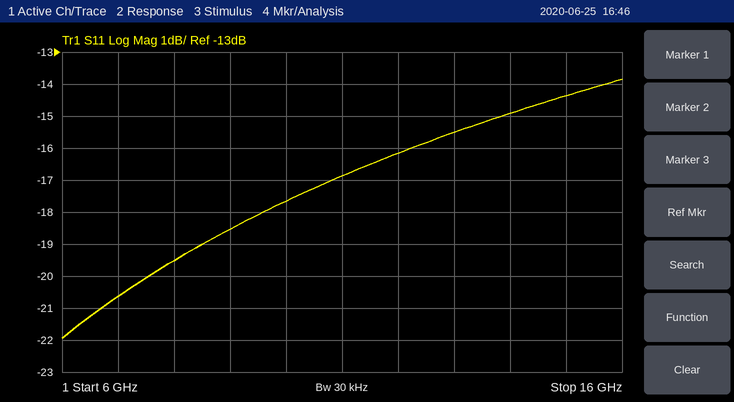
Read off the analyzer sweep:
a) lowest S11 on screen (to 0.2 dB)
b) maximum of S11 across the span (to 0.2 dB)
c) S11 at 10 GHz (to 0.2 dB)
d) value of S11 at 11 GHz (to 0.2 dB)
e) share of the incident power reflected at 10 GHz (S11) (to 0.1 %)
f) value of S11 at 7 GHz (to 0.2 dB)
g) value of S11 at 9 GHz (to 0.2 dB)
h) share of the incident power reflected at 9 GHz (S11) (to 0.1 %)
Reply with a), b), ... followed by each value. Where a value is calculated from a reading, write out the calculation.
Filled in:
a) -22.0 dB
b) -13.8 dB
c) -17.6 dB
d) -16.8 dB
e) 10^(-17.6/10) ≈ 1.7 %
f) -20.6 dB
g) -18.6 dB
h) 10^(-18.6/10) ≈ 1.4 %
